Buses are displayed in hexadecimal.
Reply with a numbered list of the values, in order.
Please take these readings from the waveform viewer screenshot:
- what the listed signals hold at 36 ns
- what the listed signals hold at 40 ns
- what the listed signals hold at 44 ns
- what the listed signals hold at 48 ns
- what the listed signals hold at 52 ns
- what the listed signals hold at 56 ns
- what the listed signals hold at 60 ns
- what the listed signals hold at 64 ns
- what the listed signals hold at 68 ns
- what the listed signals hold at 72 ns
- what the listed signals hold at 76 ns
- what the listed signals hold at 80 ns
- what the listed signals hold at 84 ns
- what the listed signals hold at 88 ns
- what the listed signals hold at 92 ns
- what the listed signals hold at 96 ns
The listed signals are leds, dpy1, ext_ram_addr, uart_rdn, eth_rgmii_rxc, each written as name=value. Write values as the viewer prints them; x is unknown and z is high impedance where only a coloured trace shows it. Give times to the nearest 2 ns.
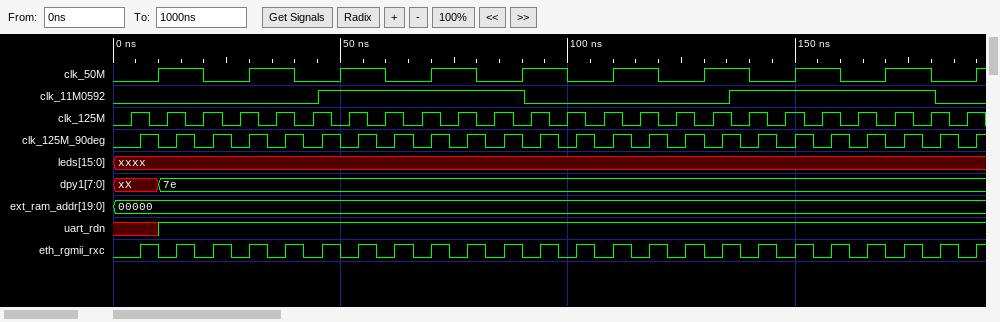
1. leds=xxxx, dpy1=7e, ext_ram_addr=00000, uart_rdn=1, eth_rgmii_rxc=0
2. leds=xxxx, dpy1=7e, ext_ram_addr=00000, uart_rdn=1, eth_rgmii_rxc=1
3. leds=xxxx, dpy1=7e, ext_ram_addr=00000, uart_rdn=1, eth_rgmii_rxc=0
4. leds=xxxx, dpy1=7e, ext_ram_addr=00000, uart_rdn=1, eth_rgmii_rxc=1
5. leds=xxxx, dpy1=7e, ext_ram_addr=00000, uart_rdn=1, eth_rgmii_rxc=0
6. leds=xxxx, dpy1=7e, ext_ram_addr=00000, uart_rdn=1, eth_rgmii_rxc=1
7. leds=xxxx, dpy1=7e, ext_ram_addr=00000, uart_rdn=1, eth_rgmii_rxc=0
8. leds=xxxx, dpy1=7e, ext_ram_addr=00000, uart_rdn=1, eth_rgmii_rxc=1
9. leds=xxxx, dpy1=7e, ext_ram_addr=00000, uart_rdn=1, eth_rgmii_rxc=0
10. leds=xxxx, dpy1=7e, ext_ram_addr=00000, uart_rdn=1, eth_rgmii_rxc=1
11. leds=xxxx, dpy1=7e, ext_ram_addr=00000, uart_rdn=1, eth_rgmii_rxc=0
12. leds=xxxx, dpy1=7e, ext_ram_addr=00000, uart_rdn=1, eth_rgmii_rxc=1
13. leds=xxxx, dpy1=7e, ext_ram_addr=00000, uart_rdn=1, eth_rgmii_rxc=0
14. leds=xxxx, dpy1=7e, ext_ram_addr=00000, uart_rdn=1, eth_rgmii_rxc=1
15. leds=xxxx, dpy1=7e, ext_ram_addr=00000, uart_rdn=1, eth_rgmii_rxc=0
16. leds=xxxx, dpy1=7e, ext_ram_addr=00000, uart_rdn=1, eth_rgmii_rxc=1
